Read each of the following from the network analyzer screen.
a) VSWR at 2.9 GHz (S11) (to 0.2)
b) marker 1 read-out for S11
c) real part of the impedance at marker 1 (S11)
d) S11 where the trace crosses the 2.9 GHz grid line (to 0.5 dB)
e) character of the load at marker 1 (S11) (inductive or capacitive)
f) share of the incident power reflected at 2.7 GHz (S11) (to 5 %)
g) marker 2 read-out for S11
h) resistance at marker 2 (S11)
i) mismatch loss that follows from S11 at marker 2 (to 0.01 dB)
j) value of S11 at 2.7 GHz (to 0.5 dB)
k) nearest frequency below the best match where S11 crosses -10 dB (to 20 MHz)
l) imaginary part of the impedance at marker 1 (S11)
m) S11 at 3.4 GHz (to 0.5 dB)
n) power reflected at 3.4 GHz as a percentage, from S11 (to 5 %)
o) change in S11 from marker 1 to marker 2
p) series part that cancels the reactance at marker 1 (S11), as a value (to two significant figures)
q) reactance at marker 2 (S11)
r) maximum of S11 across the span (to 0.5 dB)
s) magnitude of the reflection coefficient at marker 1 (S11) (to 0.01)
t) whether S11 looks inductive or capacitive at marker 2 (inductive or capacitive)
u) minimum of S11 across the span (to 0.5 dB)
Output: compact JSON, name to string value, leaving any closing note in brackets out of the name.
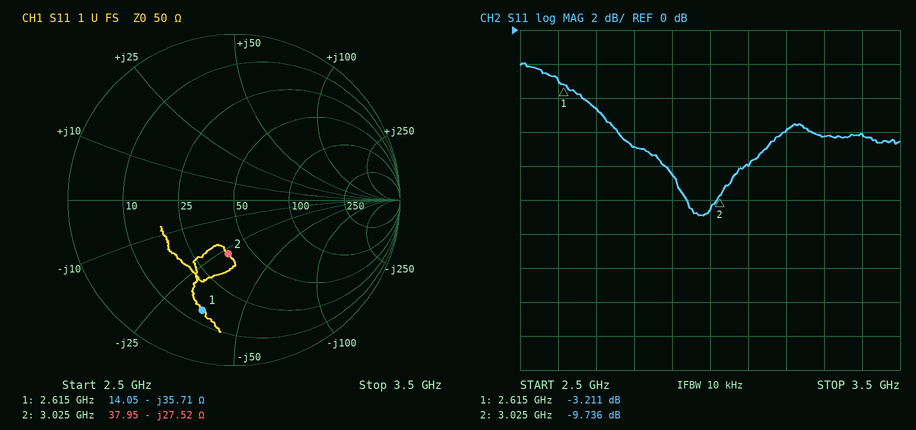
{"VSWR at 2.9 GHz (S11)": "2.2", "marker 1 read-out for S11": "-3.211 dB", "real part of the impedance at marker 1": "14.05 Ω", "S11 where the trace crosses the 2.9 GHz grid line": "-8.5 dB", "character of the load at marker 1 (S11)": "capacitive", "share of the incident power reflected at 2.7 GHz (S11)": "35 %", "marker 2 read-out for S11": "-9.736 dB", "resistance at marker 2": "37.95 Ω", "mismatch loss that follows from S11 at marker 2": "0.49 dB", "value of S11 at 2.7 GHz": "-4.5 dB", "nearest frequency below the best match where S11 crosses -10 dB": "2.94 GHz", "imaginary part of the impedance at marker 1": "-35.71 Ω", "S11 at 3.4 GHz": "-6.0 dB", "power reflected at 3.4 GHz as a percentage, from S11": "25 %", "change in S11 from marker 1 to marker 2": "-6.525 dB", "series part that cancels the reactance at marker 1 (S11), as a value": "2.2 nH", "reactance at marker 2": "-27.52 Ω", "maximum of S11 across the span": "-2.0 dB", "magnitude of the reflection coefficient at marker 1 (S11)": "0.69", "whether S11 looks inductive or capacitive at marker 2": "capacitive", "minimum of S11 across the span": "-11.0 dB"}
